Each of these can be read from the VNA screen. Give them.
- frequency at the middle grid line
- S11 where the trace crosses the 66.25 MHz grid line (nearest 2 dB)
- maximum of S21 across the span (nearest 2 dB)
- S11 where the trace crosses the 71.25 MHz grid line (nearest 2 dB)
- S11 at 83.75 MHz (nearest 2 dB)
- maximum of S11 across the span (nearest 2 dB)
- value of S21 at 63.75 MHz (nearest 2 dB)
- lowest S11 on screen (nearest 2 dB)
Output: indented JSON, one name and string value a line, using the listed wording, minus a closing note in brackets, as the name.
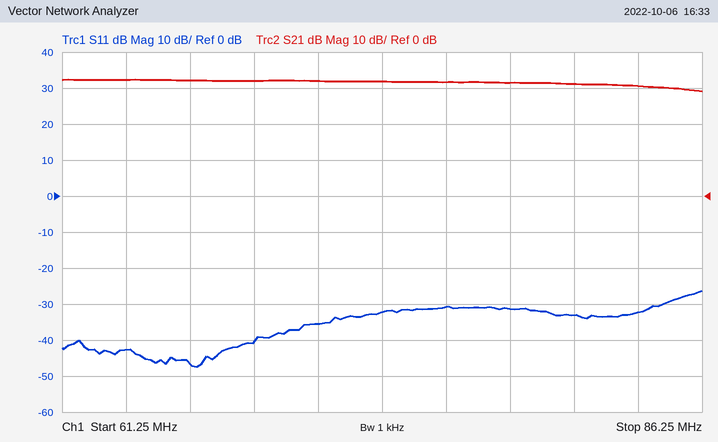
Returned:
{
  "frequency at the middle grid line": "73.75 MHz",
  "S11 where the trace crosses the 66.25 MHz grid line": "-46 dB",
  "maximum of S21 across the span": "32 dB",
  "S11 where the trace crosses the 71.25 MHz grid line": "-36 dB",
  "S11 at 83.75 MHz": "-32 dB",
  "maximum of S11 across the span": "-26 dB",
  "value of S21 at 63.75 MHz": "32 dB",
  "lowest S11 on screen": "-48 dB"
}
